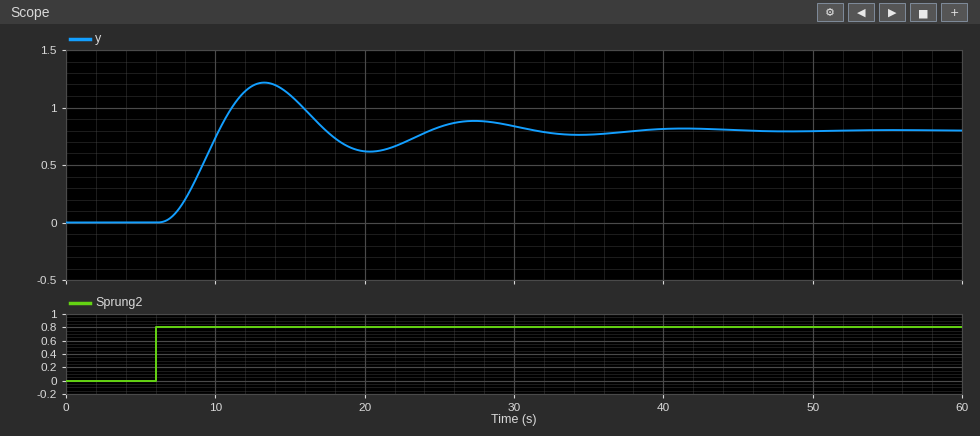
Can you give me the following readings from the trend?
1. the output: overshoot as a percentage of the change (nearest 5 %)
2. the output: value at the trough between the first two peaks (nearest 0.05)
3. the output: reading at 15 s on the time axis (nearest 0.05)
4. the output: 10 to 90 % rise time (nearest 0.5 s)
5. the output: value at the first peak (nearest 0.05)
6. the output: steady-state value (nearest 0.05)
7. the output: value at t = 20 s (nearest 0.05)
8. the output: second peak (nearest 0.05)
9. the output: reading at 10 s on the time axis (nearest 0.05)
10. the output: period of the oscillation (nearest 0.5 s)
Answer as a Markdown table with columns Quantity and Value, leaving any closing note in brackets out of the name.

| Quantity | Value |
|---|---|
| the output: overshoot as a percentage of the change | 50 % |
| the output: value at the trough between the first two peaks | 0.60 |
| the output: reading at 15 s on the time axis | 1.10 |
| the output: 10 to 90 % rise time | 2.5 s |
| the output: value at the first peak | 1.20 |
| the output: steady-state value | 0.80 |
| the output: value at t = 20 s | 0.60 |
| the output: second peak | 0.90 |
| the output: reading at 10 s on the time axis | 0.75 |
| the output: period of the oscillation | 14.0 s |
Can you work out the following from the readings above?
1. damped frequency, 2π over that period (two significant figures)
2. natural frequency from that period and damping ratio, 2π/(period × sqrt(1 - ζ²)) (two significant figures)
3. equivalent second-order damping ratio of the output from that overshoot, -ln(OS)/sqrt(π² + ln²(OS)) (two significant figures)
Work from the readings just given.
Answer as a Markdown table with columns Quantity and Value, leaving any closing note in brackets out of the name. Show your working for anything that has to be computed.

| Quantity | Value |
|---|---|
| damped frequency, 2π over that period | 2π / 14 = 0.45 rad/s |
| natural frequency from that period and damping ratio, 2π/(period × sqrt(1 - ζ²)) | 2π / (14 × sqrt(1 - 0.22²)) = 0.46 rad/s |
| equivalent second-order damping ratio of the output from that overshoot, -ln(OS)/sqrt(π² + ln²(OS)) | ln(0.5) = -0.693; 0.693 / sqrt(9.870 + 0.480) = 0.22 |
